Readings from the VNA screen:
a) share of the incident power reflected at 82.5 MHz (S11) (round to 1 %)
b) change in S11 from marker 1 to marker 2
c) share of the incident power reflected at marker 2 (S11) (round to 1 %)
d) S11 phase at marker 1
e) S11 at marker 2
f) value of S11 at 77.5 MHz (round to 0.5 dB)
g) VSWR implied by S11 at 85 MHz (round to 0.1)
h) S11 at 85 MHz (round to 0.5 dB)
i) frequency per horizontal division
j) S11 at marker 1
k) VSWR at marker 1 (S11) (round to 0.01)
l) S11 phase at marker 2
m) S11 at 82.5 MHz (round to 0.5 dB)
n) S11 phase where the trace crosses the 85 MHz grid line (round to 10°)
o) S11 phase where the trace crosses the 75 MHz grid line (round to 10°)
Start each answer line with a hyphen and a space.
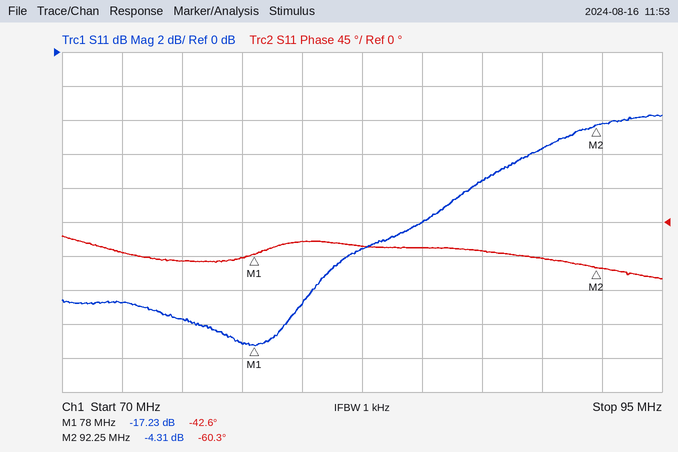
- 7 %
- 12.92 dB
- 37 %
- -42.6°
- -4.31 dB
- -17.0 dB
- 1.9
- -10.0 dB
- 2.5 MHz
- -17.23 dB
- 1.32
- -60.3°
- -11.5 dB
- -30°
- -50°
